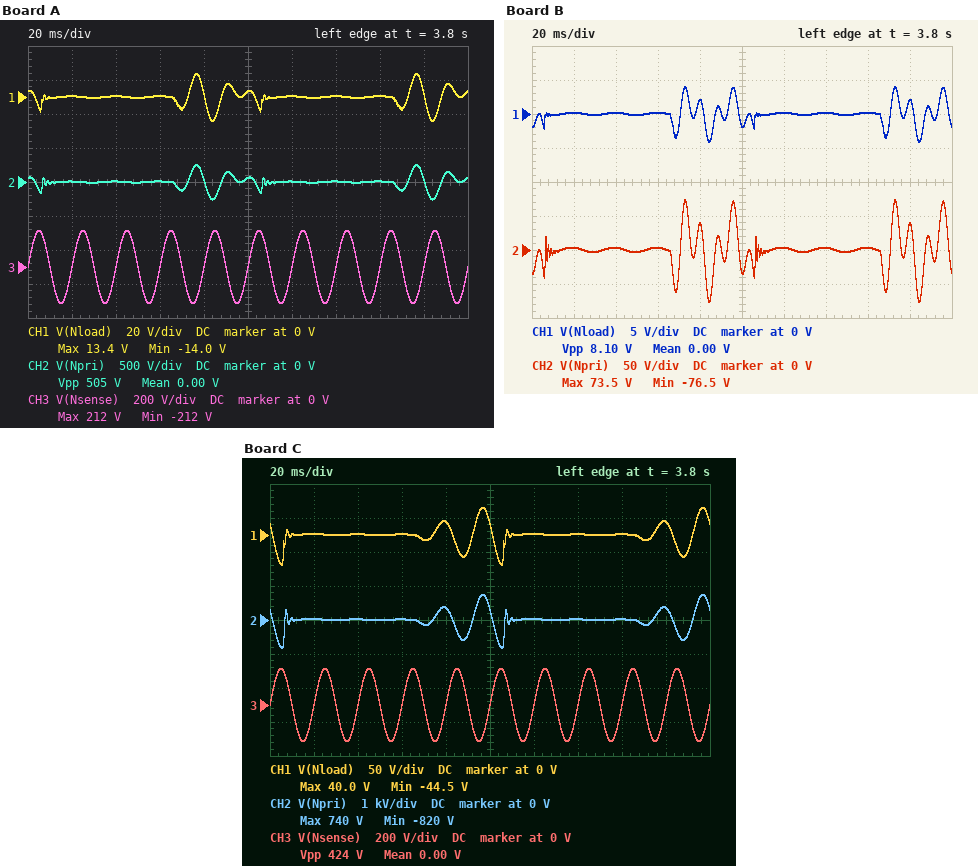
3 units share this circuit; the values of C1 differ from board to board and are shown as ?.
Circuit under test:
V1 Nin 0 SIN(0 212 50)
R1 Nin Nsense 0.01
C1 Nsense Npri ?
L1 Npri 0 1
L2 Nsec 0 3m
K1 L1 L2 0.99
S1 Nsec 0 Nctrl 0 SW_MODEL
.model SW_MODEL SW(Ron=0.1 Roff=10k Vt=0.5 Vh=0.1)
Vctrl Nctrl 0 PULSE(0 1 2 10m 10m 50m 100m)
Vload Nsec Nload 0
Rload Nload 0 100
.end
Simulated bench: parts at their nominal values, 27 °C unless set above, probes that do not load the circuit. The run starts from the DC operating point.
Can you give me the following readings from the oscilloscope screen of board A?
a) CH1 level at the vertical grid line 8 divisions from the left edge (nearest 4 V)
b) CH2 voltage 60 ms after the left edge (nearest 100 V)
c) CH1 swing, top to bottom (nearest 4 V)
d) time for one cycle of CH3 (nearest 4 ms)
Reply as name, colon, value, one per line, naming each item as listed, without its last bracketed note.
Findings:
CH1 level at the vertical grid line 8 divisions from the left edge: 0 V
CH2 voltage 60 ms after the left edge: 0 V
CH1 swing, top to bottom: 28 V
time for one cycle of CH3: 20 ms
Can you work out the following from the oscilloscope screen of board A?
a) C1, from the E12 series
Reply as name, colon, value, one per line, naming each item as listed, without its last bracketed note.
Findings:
C1, from the E12 series: 3.9 µF
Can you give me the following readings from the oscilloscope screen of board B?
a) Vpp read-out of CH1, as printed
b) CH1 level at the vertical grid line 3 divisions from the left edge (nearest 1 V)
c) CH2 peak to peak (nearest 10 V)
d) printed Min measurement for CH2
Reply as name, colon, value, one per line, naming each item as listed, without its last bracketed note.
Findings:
Vpp read-out of CH1, as printed: 8.10 V
CH1 level at the vertical grid line 3 divisions from the left edge: 0 V
CH2 peak to peak: 150 V
printed Min measurement for CH2: -76.5 V
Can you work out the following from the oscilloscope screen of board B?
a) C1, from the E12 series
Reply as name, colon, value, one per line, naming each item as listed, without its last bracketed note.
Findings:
C1, from the E12 series: 1.5 µF
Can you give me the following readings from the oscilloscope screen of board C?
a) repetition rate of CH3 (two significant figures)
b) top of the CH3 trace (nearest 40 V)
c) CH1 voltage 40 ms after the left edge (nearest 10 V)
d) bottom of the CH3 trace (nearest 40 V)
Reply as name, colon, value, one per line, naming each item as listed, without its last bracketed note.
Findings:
repetition rate of CH3: 50 Hz
top of the CH3 trace: 200 V
CH1 voltage 40 ms after the left edge: 0 V
bottom of the CH3 trace: -200 V
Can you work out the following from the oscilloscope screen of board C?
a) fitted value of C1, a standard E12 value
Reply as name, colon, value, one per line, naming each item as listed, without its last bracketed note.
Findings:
fitted value of C1, a standard E12 value: 6.8 µF
